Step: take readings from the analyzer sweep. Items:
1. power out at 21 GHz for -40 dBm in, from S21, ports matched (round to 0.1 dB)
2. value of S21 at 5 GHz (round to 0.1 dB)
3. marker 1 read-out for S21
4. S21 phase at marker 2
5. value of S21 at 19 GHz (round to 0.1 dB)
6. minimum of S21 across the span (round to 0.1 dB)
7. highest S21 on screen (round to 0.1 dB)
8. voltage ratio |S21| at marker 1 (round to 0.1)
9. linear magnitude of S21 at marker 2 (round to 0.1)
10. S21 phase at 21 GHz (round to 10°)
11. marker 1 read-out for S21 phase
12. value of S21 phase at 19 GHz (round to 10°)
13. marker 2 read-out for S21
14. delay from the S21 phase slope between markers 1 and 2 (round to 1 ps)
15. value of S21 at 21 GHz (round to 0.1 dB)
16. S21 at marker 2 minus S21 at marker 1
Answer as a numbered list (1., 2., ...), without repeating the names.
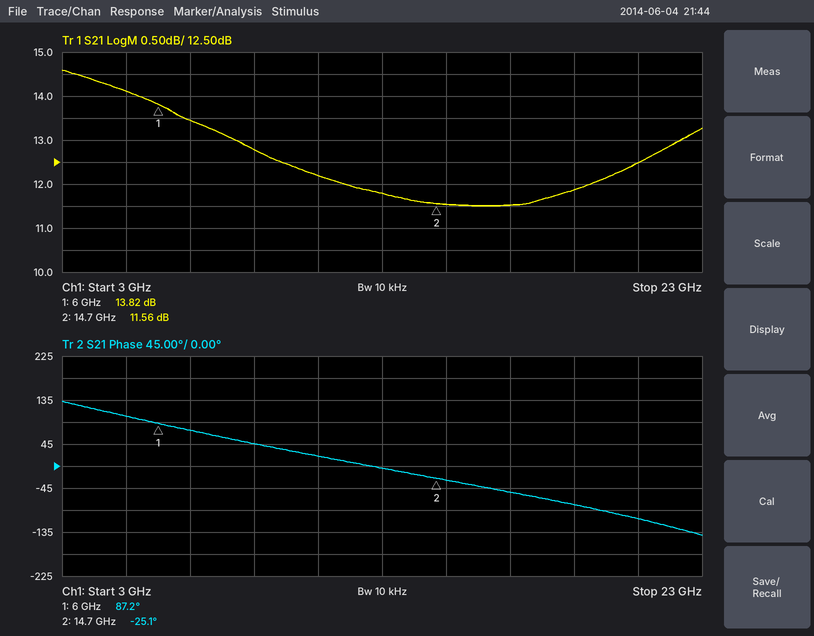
1. -27.5 dBm
2. 14.1 dB
3. 13.82 dB
4. -25.1°
5. 11.9 dB
6. 11.5 dB
7. 14.6 dB
8. 4.9
9. 3.8
10. -110°
11. 87.2°
12. -80°
13. 11.56 dB
14. 36 ps
15. 12.5 dB
16. -2.26 dB
